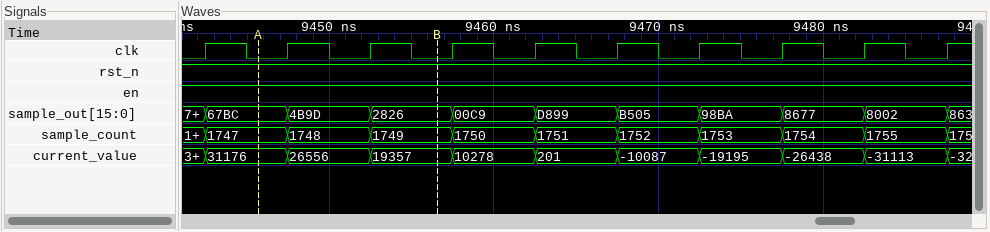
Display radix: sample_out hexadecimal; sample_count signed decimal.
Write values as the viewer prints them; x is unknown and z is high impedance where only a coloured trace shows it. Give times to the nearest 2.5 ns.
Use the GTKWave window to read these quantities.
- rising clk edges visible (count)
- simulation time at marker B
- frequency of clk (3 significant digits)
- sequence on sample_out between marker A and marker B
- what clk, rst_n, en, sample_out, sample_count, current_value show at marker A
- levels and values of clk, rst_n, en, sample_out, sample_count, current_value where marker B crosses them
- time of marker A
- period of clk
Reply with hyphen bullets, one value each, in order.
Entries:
- 10
- 9457.5 ns
- 200 MHz
- 67BC, 4B9D, 2826
- clk=0, rst_n=1, en=1, sample_out=67BC, sample_count=1747, current_value=31176
- clk=0, rst_n=1, en=1, sample_out=2826, sample_count=1749, current_value=19357
- 9445 ns
- 5 ns
